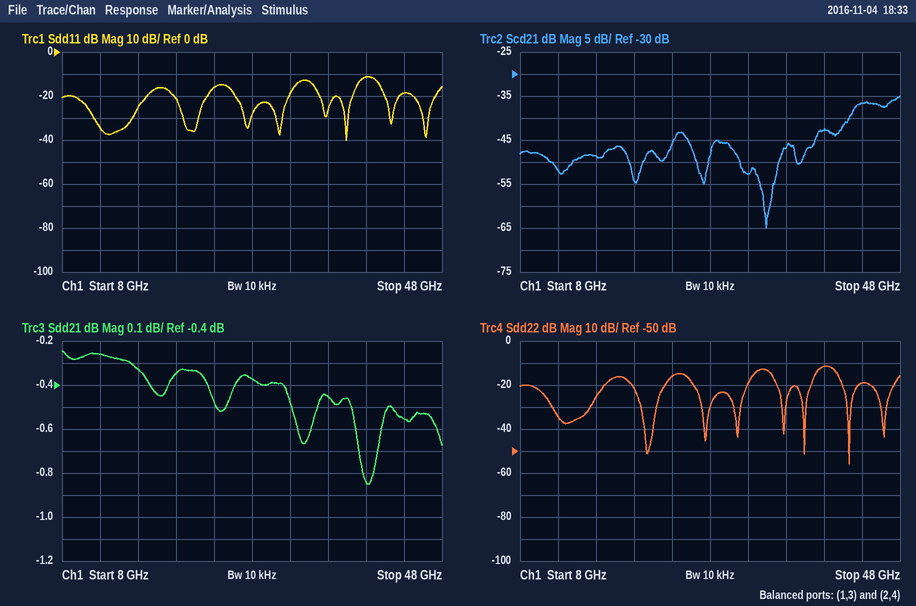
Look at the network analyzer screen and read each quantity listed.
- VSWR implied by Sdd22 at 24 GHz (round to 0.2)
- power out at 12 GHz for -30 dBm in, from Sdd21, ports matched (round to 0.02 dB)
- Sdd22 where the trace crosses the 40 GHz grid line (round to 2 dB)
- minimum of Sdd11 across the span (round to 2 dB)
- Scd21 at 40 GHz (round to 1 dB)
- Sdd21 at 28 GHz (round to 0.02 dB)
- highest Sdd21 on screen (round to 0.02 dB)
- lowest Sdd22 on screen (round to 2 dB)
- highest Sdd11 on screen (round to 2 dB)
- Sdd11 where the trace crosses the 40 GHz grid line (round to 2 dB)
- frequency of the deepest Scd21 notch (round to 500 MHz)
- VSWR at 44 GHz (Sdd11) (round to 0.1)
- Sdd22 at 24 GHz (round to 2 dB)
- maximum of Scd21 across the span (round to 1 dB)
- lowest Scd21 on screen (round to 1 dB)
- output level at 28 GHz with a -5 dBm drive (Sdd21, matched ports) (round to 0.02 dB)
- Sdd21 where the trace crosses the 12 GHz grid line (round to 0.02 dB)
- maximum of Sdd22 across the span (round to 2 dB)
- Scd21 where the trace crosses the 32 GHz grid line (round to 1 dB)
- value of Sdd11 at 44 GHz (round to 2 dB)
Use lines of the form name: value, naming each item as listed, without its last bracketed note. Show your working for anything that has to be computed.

VSWR implied by Sdd22 at 24 GHz: |Γ| = 10^(-16/20) = 0.1585; VSWR = (1 + 0.1585)/(1 − 0.1585) ≈ 1.4
power out at 12 GHz for -30 dBm in, from Sdd21, ports matched: -30 dBm + (-0.26 dB) = -30.26 dBm
Sdd22 where the trace crosses the 40 GHz grid line: -12 dB
minimum of Sdd11 across the span: -40 dB
Scd21 at 40 GHz: -43 dB
Sdd21 at 28 GHz: -0.38 dB
highest Sdd21 on screen: -0.24 dB
lowest Sdd22 on screen: -56 dB
highest Sdd11 on screen: -12 dB
Sdd11 where the trace crosses the 40 GHz grid line: -12 dB
frequency of the deepest Scd21 notch: 34.0 GHz
VSWR at 44 GHz (Sdd11): |Γ| = 10^(-18/20) = 0.1259; VSWR = (1 + 0.1259)/(1 − 0.1259) ≈ 1.3
Sdd22 at 24 GHz: -16 dB
maximum of Scd21 across the span: -35 dB
lowest Scd21 on screen: -65 dB
output level at 28 GHz with a -5 dBm drive (Sdd21, matched ports): -5 dBm + (-0.38 dB) = -5.38 dBm
Sdd21 where the trace crosses the 12 GHz grid line: -0.26 dB
maximum of Sdd22 across the span: -12 dB
Scd21 where the trace crosses the 32 GHz grid line: -53 dB
value of Sdd11 at 44 GHz: -18 dB
